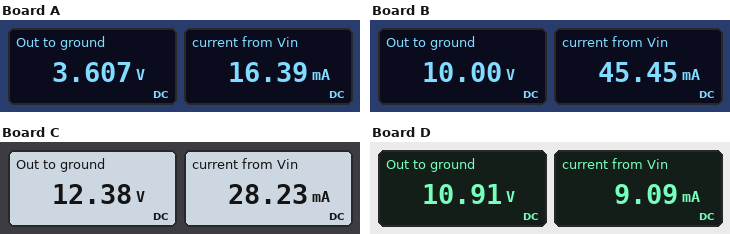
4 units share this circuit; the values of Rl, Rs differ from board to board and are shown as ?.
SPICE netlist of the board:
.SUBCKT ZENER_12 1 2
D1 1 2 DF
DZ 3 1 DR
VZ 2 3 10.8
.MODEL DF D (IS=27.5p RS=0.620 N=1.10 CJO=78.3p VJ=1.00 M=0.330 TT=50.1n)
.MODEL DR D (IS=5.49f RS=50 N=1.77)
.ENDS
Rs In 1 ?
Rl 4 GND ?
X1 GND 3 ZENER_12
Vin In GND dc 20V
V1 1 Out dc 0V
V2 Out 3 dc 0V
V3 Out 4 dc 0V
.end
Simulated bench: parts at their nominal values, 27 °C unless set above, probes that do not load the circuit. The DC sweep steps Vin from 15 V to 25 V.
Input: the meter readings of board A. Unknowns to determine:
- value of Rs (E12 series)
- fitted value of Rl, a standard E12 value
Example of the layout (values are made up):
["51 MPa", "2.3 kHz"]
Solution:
["1 kΩ", "220 Ω"]
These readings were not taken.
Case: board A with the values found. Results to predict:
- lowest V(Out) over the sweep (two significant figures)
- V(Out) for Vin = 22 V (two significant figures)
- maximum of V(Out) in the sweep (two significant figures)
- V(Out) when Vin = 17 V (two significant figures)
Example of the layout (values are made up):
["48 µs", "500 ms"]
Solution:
["2.7 V", "4.0 V", "4.5 V", "3.1 V"]
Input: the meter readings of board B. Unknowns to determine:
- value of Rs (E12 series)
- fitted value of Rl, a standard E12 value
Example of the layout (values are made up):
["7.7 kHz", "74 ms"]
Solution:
["220 Ω", "220 Ω"]
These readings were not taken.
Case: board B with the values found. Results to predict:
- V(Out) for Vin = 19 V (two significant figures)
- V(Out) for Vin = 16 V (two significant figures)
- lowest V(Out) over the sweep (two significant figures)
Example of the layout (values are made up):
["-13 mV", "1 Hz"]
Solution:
["9.5 V", "8.0 V", "7.5 V"]
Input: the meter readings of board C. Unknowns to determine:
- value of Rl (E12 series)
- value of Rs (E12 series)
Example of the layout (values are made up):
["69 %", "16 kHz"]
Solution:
["560 Ω", "270 Ω"]
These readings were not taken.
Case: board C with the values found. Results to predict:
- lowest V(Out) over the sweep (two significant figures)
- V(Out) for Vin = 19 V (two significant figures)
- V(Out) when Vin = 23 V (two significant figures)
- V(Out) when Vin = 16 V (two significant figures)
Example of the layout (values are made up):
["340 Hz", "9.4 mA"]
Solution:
["10 V", "12 V", "13 V", "11 V"]
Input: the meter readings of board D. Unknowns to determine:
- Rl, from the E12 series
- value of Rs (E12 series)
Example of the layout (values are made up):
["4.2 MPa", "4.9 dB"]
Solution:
["1.2 kΩ", "1 kΩ"]
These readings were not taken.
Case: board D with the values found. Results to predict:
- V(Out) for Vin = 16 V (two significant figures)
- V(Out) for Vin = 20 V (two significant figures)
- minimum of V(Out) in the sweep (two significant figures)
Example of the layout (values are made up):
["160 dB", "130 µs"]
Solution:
["8.7 V", "11 V", "8.2 V"]
